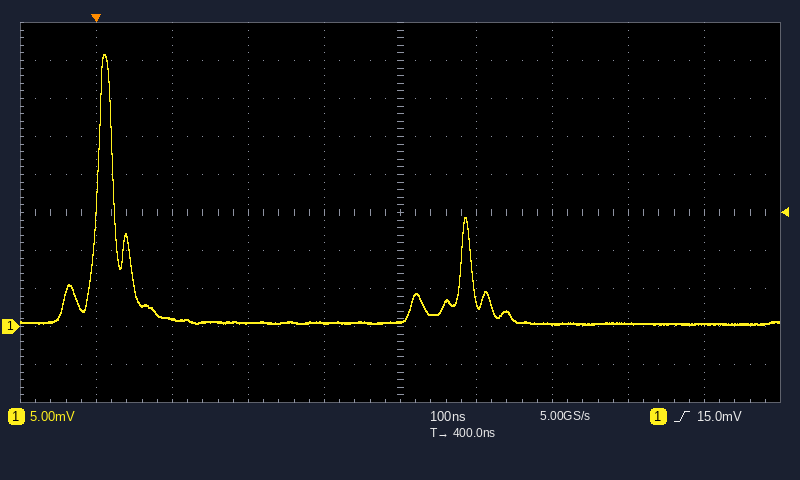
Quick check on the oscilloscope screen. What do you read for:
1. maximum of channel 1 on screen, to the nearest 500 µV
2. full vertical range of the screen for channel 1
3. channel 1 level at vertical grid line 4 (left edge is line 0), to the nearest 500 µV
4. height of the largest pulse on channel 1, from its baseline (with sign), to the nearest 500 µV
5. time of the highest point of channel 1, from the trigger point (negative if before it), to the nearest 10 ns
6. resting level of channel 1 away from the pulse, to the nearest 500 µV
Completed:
36.0 mV
50 mV
500 µV
+35.5 mV
+10 ns
500 µV
